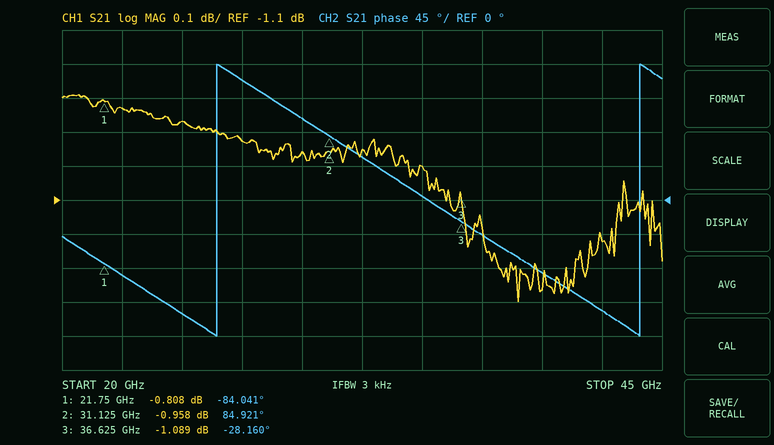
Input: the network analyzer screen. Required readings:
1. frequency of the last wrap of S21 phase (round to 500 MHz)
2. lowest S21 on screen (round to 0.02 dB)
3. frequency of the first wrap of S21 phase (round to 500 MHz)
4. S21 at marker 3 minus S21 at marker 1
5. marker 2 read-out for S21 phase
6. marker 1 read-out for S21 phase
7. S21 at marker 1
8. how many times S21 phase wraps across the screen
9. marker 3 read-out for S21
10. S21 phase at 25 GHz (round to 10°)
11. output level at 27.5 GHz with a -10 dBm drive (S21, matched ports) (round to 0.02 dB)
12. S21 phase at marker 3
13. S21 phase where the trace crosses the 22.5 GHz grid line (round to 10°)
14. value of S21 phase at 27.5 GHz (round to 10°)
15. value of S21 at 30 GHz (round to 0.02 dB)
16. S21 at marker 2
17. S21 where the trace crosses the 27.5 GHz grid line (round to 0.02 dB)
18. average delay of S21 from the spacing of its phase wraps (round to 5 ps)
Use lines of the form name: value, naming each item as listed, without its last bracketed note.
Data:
frequency of the last wrap of S21 phase: 44.0 GHz
lowest S21 on screen: -1.40 dB
frequency of the first wrap of S21 phase: 26.5 GHz
S21 at marker 3 minus S21 at marker 1: -0.281 dB
marker 2 read-out for S21 phase: 84.921°
marker 1 read-out for S21 phase: -84.041°
S21 at marker 1: -0.808 dB
how many times S21 phase wraps across the screen: 2
marker 3 read-out for S21: -1.089 dB
S21 phase at 25 GHz: -150°
output level at 27.5 GHz with a -10 dBm drive (S21, matched ports): -10.92 dBm
S21 phase at marker 3: -28.160°
S21 phase where the trace crosses the 22.5 GHz grid line: -100°
value of S21 phase at 27.5 GHz: 160°
value of S21 at 30 GHz: -0.96 dB
S21 at marker 2: -0.958 dB
S21 where the trace crosses the 27.5 GHz grid line: -0.92 dB
average delay of S21 from the spacing of its phase wraps: 55 ps
